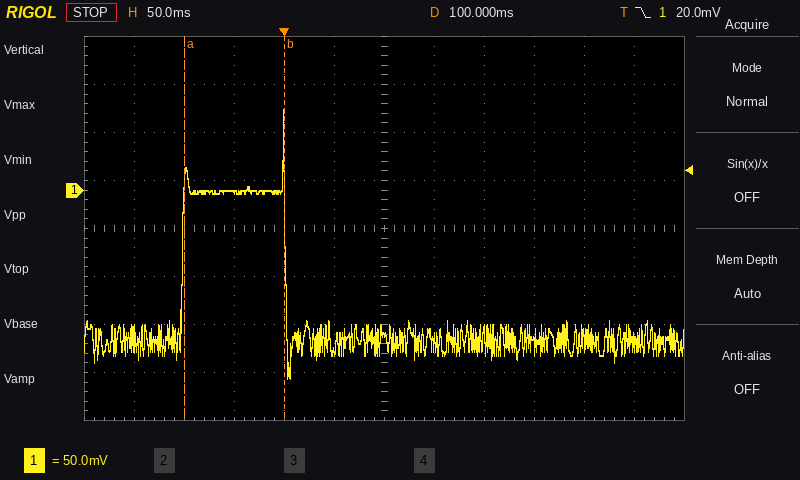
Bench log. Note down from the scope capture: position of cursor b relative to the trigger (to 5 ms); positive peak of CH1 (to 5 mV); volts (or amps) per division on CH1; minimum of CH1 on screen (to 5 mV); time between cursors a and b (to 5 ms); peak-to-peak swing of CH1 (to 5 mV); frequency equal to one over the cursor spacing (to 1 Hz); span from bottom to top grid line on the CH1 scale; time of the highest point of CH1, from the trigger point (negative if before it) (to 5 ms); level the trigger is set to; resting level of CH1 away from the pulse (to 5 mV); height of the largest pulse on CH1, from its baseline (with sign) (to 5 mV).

0 ms
85 mV
50 mV
-195 mV
100 ms
280 mV
10 Hz
400 mV
0 ms
20.0 mV
-155 mV
+240 mV
